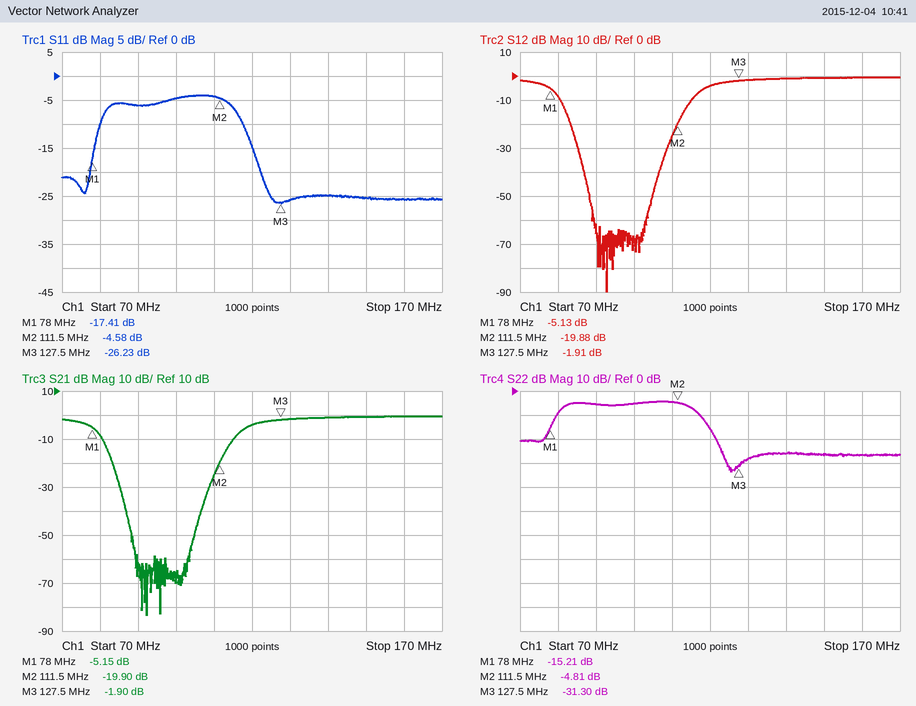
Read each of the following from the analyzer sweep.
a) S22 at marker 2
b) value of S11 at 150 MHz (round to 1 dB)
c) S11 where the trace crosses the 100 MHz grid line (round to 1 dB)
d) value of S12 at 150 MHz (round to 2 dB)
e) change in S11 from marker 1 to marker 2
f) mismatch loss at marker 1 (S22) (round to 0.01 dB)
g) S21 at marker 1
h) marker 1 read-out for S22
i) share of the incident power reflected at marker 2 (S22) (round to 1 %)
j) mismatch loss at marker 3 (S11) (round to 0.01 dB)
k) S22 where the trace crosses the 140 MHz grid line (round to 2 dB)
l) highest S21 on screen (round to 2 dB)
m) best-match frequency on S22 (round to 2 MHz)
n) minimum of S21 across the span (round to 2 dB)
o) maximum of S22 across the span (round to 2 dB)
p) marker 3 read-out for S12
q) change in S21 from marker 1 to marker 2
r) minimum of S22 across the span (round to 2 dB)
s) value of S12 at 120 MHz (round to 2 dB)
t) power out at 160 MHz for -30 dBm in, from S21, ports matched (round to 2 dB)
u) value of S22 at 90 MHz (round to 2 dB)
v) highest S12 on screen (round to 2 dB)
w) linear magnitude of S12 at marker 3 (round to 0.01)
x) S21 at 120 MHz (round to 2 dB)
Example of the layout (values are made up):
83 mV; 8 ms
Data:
-4.81 dB; -25 dB; -5 dB; 0 dB; 12.83 dB; 0.13 dB; -5.15 dB; -15.21 dB; 33 %; 0.01 dB; -26 dB; 0 dB; 126 MHz; -84 dB; -4 dB; -1.91 dB; -14.75 dB; -34 dB; -4 dB; -30 dBm; -6 dB; 0 dB; 0.80; -4 dB
